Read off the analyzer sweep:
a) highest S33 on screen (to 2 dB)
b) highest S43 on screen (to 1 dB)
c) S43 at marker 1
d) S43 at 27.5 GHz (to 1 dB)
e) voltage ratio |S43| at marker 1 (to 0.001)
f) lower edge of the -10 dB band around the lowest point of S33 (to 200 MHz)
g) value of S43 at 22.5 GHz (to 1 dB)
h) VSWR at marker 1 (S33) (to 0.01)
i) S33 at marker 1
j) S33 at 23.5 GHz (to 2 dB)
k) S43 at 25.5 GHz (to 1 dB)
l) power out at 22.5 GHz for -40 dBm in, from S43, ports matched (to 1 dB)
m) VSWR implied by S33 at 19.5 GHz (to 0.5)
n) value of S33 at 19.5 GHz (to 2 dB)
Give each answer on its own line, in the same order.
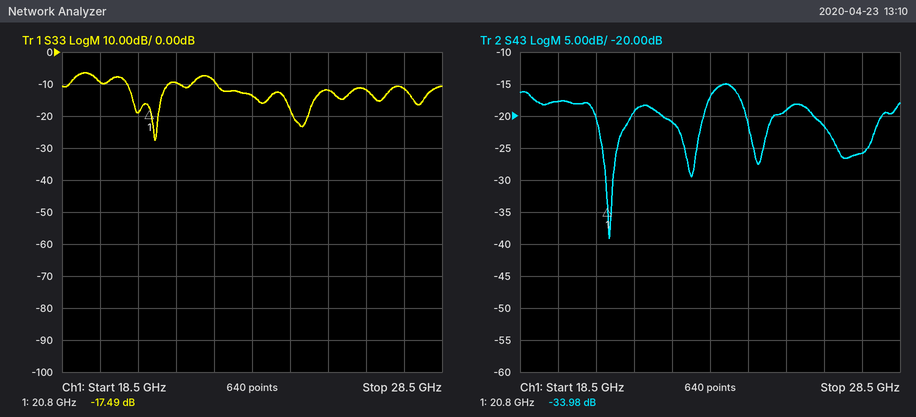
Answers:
-6 dB
-15 dB
-33.98 dB
-26 dB
0.020
20.2 GHz
-21 dB
1.31
-17.49 dB
-14 dB
-19 dB
-61 dBm
2.0
-10 dB
